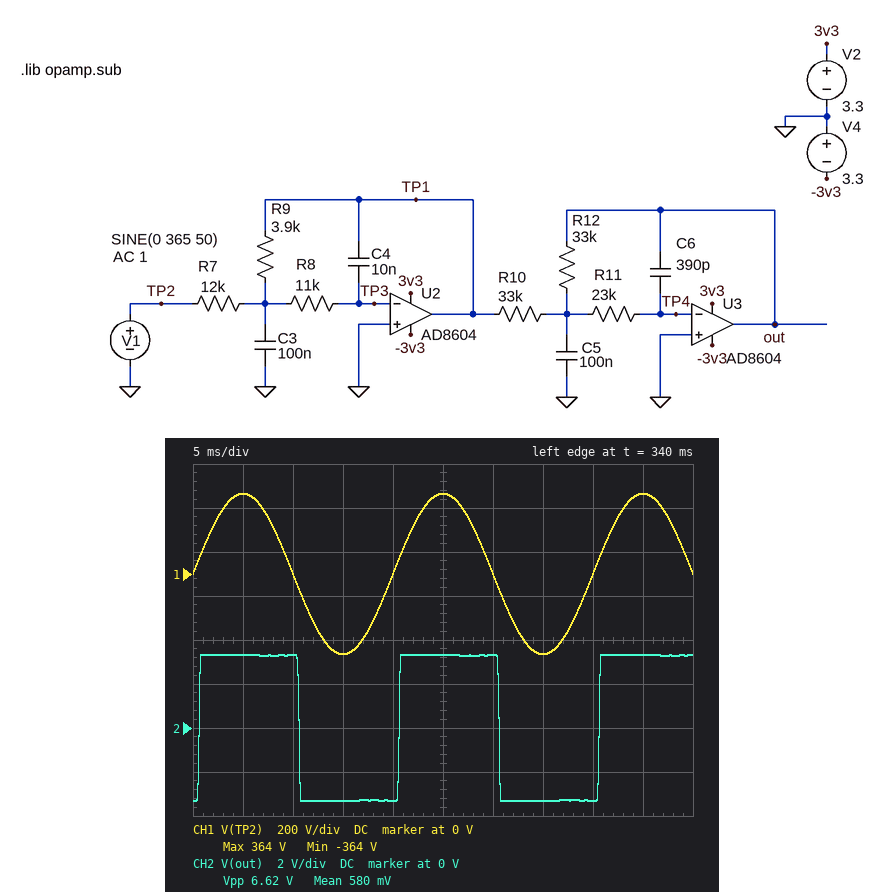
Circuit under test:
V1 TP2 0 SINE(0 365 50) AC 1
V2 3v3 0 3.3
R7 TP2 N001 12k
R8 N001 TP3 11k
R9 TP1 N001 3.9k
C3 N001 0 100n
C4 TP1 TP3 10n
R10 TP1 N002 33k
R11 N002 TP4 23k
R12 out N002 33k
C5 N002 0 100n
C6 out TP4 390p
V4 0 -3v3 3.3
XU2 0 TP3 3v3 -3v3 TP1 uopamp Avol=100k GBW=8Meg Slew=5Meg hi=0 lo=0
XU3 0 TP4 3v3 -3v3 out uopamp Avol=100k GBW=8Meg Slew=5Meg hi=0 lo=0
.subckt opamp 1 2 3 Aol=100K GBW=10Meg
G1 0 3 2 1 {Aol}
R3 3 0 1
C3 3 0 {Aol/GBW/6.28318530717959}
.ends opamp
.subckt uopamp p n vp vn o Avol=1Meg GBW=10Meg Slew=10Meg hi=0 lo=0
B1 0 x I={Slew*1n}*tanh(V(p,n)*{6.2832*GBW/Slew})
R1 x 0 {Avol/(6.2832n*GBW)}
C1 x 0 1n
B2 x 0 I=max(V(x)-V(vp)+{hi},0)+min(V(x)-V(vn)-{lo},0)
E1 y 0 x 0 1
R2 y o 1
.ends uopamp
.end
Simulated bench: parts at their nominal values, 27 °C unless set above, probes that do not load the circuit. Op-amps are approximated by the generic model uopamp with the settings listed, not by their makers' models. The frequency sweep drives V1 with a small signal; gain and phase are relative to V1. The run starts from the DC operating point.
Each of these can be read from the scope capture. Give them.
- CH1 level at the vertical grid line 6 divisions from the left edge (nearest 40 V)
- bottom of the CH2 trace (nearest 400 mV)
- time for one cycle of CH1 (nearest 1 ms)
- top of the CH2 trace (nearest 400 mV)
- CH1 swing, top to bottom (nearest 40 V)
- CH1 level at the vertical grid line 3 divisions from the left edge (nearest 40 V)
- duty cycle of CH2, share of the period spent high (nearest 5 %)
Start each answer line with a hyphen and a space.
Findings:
- 0 V
- -3.2 V
- 20 ms
- 3.2 V
- 720 V
- -360 V
- 50 %
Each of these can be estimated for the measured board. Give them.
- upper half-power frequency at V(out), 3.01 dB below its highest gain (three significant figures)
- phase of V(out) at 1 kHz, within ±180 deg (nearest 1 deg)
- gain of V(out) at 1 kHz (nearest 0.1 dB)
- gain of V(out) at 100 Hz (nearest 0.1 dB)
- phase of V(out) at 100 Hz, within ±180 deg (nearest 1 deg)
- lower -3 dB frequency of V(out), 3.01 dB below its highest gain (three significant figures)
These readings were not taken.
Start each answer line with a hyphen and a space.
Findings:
- 976 Hz
- 108 deg
- -0.6 dB
- -9.6 dB
- -8 deg
- 789 Hz
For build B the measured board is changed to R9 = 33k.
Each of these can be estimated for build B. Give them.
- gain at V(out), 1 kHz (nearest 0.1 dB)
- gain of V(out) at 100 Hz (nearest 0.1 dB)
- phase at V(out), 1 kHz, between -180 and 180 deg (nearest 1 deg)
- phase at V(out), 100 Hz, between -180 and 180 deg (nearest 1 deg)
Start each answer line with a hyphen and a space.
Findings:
- -2.5 dB
- 9.1 dB
- 68 deg
- -30 deg
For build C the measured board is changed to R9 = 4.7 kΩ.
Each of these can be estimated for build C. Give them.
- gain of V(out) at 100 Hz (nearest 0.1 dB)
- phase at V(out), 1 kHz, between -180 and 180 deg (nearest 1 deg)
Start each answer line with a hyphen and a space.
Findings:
- -7.9 dB
- 99 deg
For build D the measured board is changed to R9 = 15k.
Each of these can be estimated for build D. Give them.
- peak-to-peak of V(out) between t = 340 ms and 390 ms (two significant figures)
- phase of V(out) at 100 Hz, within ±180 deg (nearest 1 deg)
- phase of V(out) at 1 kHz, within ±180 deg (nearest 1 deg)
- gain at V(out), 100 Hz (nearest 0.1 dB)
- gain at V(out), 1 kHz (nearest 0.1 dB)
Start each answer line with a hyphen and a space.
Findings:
- 6.6 V
- -16 deg
- 73 deg
- 2.3 dB
- -2.0 dB
